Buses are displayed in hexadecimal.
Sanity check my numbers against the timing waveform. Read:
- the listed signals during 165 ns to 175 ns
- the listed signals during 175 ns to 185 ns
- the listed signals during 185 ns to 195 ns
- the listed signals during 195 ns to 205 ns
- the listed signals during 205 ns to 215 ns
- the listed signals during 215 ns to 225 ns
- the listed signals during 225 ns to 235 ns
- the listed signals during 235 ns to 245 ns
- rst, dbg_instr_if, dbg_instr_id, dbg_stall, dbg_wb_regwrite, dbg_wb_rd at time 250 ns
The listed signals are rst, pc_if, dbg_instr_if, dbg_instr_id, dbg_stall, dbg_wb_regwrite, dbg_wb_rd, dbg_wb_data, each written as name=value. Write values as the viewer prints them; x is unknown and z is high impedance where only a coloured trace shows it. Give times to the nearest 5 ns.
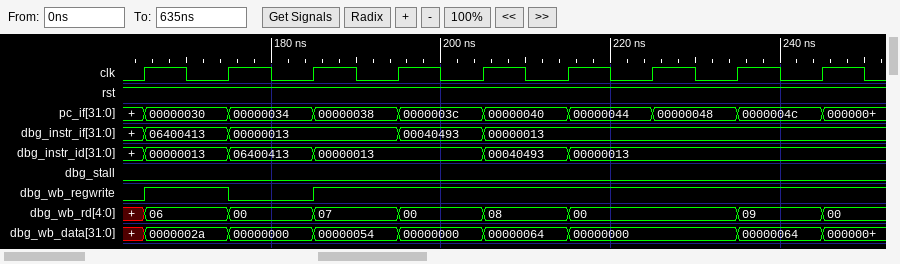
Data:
rst=1, pc_if=00000030, dbg_instr_if=06400413, dbg_instr_id=00000013, dbg_stall=0, dbg_wb_regwrite=1, dbg_wb_rd=06, dbg_wb_data=0000002a
rst=1, pc_if=00000034, dbg_instr_if=00000013, dbg_instr_id=06400413, dbg_stall=0, dbg_wb_regwrite=0, dbg_wb_rd=00, dbg_wb_data=00000000
rst=1, pc_if=00000038, dbg_instr_if=00000013, dbg_instr_id=00000013, dbg_stall=0, dbg_wb_regwrite=1, dbg_wb_rd=07, dbg_wb_data=00000054
rst=1, pc_if=0000003c, dbg_instr_if=00040493, dbg_instr_id=00000013, dbg_stall=0, dbg_wb_regwrite=1, dbg_wb_rd=00, dbg_wb_data=00000000
rst=1, pc_if=00000040, dbg_instr_if=00000013, dbg_instr_id=00040493, dbg_stall=0, dbg_wb_regwrite=1, dbg_wb_rd=08, dbg_wb_data=00000064
rst=1, pc_if=00000044, dbg_instr_if=00000013, dbg_instr_id=00000013, dbg_stall=0, dbg_wb_regwrite=1, dbg_wb_rd=00, dbg_wb_data=00000000
rst=1, pc_if=00000048, dbg_instr_if=00000013, dbg_instr_id=00000013, dbg_stall=0, dbg_wb_regwrite=1, dbg_wb_rd=00, dbg_wb_data=00000000
rst=1, pc_if=0000004c, dbg_instr_if=00000013, dbg_instr_id=00000013, dbg_stall=0, dbg_wb_regwrite=1, dbg_wb_rd=09, dbg_wb_data=00000064
rst=1, dbg_instr_if=00000013, dbg_instr_id=00000013, dbg_stall=0, dbg_wb_regwrite=1, dbg_wb_rd=00
